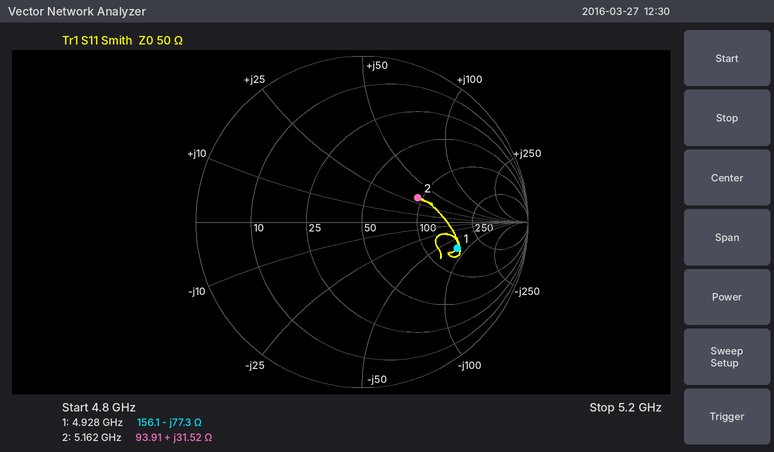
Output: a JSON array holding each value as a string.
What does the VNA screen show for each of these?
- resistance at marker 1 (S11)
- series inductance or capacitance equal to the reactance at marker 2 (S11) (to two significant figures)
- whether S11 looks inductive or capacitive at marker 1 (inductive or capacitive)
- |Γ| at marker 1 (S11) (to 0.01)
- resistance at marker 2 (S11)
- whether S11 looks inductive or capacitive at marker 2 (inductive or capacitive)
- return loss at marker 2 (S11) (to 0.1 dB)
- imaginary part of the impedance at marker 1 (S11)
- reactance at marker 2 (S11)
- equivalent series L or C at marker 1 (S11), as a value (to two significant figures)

["156.1 Ω", "970 pH", "capacitive", "0.60", "93.91 Ω", "inductive", "8.7 dB", "-77.3 Ω", "+31.52 Ω", "420 fF"]
